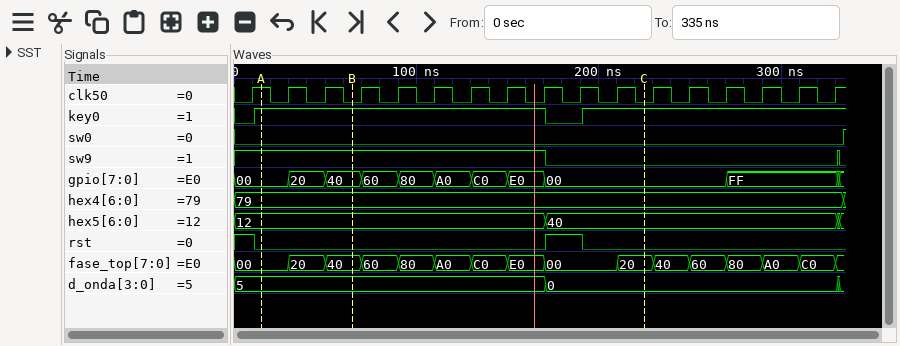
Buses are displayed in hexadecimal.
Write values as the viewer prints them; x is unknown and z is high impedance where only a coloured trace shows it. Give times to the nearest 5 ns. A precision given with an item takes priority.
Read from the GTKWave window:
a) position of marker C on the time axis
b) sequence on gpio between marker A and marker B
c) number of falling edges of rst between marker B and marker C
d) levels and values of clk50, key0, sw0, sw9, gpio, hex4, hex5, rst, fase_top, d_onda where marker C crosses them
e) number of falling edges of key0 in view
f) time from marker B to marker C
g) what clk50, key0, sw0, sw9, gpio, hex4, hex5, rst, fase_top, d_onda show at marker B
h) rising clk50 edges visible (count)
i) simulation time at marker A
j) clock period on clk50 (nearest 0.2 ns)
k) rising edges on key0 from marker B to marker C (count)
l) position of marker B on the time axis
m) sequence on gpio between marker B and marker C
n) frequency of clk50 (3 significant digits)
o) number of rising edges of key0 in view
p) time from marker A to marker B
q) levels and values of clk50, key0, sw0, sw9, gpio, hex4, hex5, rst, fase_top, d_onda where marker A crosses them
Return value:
225 ns
00, 20, 40
1
clk50=0, key0=1, sw0=0, sw9=0, gpio=00, hex4=79, hex5=40, rst=0, fase_top=20, d_onda=0
1
160 ns
clk50=0, key0=1, sw0=0, sw9=1, gpio=40, hex4=79, hex5=12, rst=0, fase_top=40, d_onda=5
17
15 ns
20 ns
1
65 ns
40, 60, 80, A0, C0, E0, 00
50.0 MHz
2
50 ns
clk50=1, key0=1, sw0=0, sw9=1, gpio=00, hex4=79, hex5=12, rst=0, fase_top=00, d_onda=5
